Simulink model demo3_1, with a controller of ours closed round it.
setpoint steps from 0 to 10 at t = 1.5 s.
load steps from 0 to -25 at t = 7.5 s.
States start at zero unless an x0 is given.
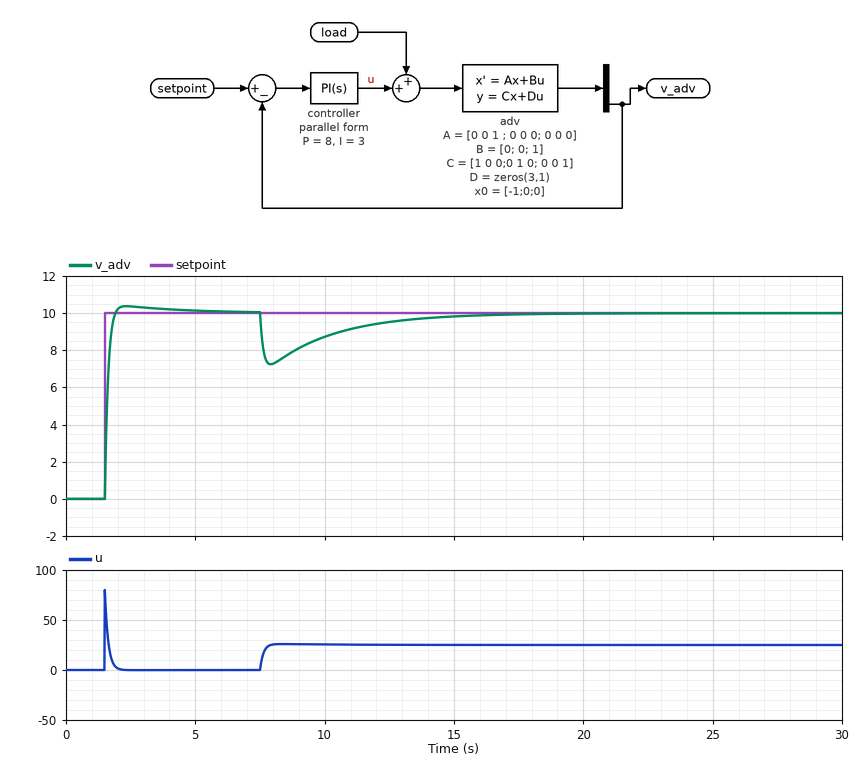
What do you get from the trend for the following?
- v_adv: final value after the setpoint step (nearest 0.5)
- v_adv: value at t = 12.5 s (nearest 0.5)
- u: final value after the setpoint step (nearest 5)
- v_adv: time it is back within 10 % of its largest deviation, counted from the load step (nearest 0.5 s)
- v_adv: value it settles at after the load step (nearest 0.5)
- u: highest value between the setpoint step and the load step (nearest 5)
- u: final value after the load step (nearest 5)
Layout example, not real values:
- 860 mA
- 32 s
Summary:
- 10.0
- 9.5
- 0
- 6.5 s
- 10.0
- 80
- 25
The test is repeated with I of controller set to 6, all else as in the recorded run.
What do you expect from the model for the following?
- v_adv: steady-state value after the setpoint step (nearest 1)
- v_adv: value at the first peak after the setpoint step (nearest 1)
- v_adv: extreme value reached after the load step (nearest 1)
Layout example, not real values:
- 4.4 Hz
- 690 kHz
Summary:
- 10
- 11
- 7
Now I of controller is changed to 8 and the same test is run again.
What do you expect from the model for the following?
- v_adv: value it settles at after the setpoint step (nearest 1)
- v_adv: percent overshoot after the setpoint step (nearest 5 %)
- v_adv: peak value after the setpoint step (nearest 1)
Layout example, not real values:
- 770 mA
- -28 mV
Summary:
- 10
- 10 %
- 11
